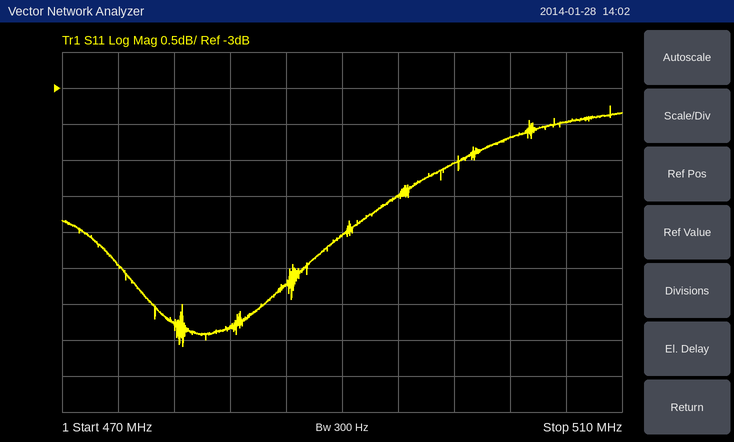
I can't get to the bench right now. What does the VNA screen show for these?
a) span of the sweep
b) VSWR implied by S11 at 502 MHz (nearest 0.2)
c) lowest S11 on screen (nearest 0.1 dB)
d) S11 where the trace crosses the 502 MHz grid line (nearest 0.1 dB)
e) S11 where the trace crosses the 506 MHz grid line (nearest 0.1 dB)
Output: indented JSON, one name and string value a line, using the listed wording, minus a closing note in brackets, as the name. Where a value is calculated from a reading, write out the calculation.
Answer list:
{
  "span of the sweep": "40 MHz",
  "VSWR implied by S11 at 502 MHz": "|Γ| = 10^(-3.7/20) = 0.6531; VSWR = (1 + 0.6531)/(1 − 0.6531) ≈ 4.8",
  "lowest S11 on screen": "-6.6 dB",
  "S11 where the trace crosses the 502 MHz grid line": "-3.7 dB",
  "S11 where the trace crosses the 506 MHz grid line": "-3.5 dB"
}
